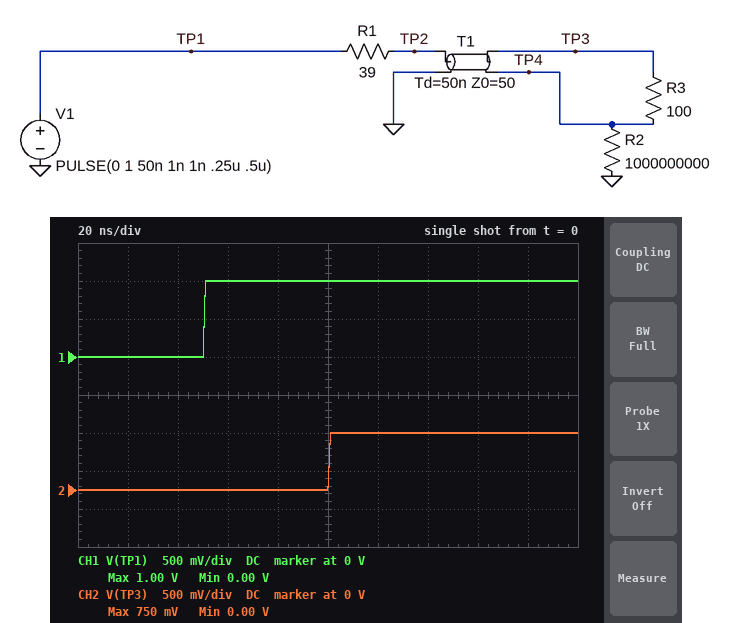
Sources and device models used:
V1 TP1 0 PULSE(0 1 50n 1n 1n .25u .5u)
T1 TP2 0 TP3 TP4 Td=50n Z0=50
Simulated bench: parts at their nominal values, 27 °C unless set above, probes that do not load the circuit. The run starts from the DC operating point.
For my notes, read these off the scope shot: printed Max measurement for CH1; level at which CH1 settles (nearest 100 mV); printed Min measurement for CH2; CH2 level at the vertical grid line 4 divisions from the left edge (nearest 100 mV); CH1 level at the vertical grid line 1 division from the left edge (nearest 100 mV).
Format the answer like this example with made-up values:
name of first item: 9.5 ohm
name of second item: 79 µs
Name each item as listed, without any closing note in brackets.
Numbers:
printed Max measurement for CH1: 1.00 V
level at which CH1 settles: 1.0 V
printed Min measurement for CH2: 0.00 V
CH2 level at the vertical grid line 4 divisions from the left edge: 0 V
CH1 level at the vertical grid line 1 division from the left edge: 0 V
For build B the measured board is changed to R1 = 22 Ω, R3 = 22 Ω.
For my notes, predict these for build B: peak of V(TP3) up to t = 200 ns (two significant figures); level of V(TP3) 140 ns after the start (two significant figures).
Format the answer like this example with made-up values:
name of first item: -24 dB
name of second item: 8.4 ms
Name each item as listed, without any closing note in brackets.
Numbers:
peak of V(TP3) up to t = 200 ns: 430 mV
level of V(TP3) 140 ns after the start: 420 mV
